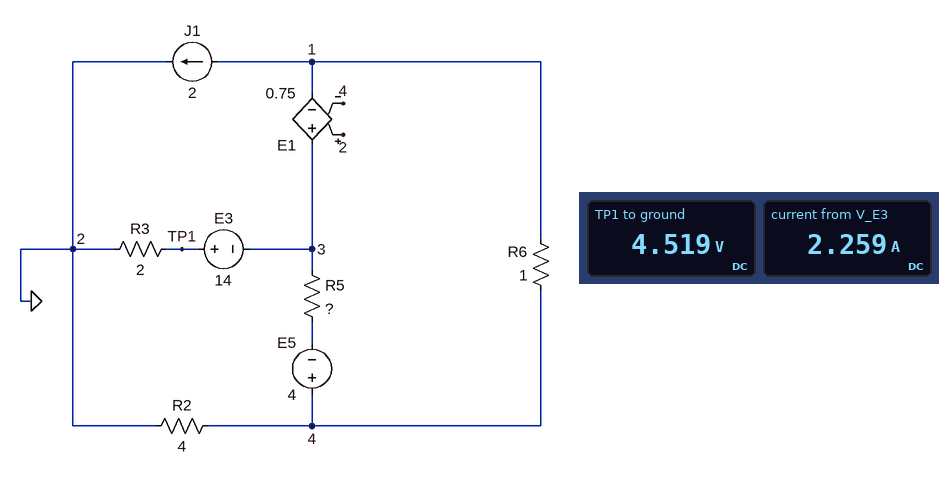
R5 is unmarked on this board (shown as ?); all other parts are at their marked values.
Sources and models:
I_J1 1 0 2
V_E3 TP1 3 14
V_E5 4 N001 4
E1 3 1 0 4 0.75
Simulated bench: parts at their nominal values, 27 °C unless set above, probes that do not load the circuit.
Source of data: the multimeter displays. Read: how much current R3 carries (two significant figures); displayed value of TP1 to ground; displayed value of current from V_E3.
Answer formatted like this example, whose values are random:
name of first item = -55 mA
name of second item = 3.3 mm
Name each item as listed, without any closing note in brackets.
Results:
how much current R3 carries = 2.3 A
displayed value of TP1 to ground = 4.519 V
displayed value of current from V_E3 = 2.259 A
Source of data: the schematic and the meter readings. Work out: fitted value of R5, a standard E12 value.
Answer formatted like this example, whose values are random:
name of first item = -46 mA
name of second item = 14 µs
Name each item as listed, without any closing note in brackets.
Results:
fitted value of R5, a standard E12 value = 12 Ω
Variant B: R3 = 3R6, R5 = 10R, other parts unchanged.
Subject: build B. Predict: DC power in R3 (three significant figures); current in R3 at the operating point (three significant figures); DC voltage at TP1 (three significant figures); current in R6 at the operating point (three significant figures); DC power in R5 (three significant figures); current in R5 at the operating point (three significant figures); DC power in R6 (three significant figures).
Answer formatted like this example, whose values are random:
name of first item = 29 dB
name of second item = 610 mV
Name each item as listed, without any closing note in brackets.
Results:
DC power in R3 = 9.26 W
current in R3 at the operating point = 1.60 A
DC voltage at TP1 = 5.77 V
current in R6 at the operating point = 4.62 A
DC power in R5 = 10.4 W
current in R5 at the operating point = 1.02 A
DC power in R6 = 21.4 W
